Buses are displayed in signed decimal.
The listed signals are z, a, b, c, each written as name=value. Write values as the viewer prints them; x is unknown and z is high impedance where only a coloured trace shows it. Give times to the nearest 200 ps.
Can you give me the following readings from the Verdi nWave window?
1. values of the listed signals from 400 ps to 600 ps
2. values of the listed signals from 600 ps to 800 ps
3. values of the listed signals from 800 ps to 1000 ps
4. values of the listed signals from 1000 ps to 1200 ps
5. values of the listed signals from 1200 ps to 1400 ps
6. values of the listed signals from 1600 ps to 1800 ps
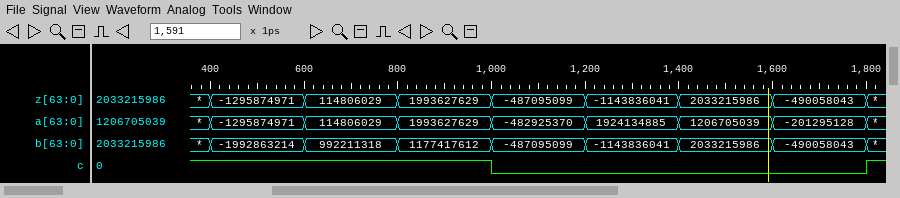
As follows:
z=-1295874971, a=-1295874971, b=-1992863214, c=1
z=114806029, a=114806029, b=992211318, c=1
z=1993627629, a=1993627629, b=1177417612, c=1
z=-487095099, a=-482925370, b=-487095099, c=0
z=-1143836041, a=1924134885, b=-1143836041, c=0
z=-490058043, a=-201295128, b=-490058043, c=0
